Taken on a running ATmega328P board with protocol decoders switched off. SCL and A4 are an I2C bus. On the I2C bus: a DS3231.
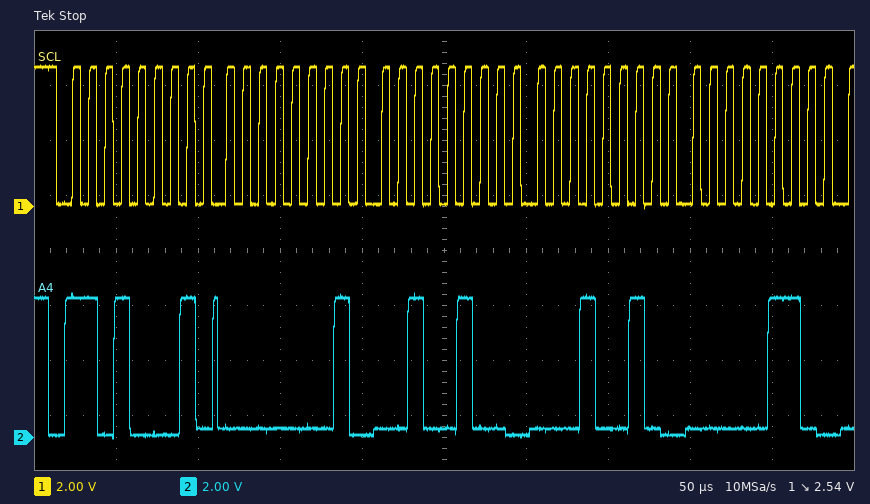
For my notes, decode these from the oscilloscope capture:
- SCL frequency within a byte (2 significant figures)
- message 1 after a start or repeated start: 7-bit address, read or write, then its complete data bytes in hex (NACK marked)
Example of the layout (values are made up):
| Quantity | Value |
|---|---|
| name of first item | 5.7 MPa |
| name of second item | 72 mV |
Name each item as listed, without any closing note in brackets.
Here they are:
| Quantity | Value |
|---|---|
| SCL frequency within a byte | 100 kHz |
| message 1 after a start or repeated start: 7-bit address, read or write, then its complete data bytes in hex | 0x68 read: 01 24 12 06 |
